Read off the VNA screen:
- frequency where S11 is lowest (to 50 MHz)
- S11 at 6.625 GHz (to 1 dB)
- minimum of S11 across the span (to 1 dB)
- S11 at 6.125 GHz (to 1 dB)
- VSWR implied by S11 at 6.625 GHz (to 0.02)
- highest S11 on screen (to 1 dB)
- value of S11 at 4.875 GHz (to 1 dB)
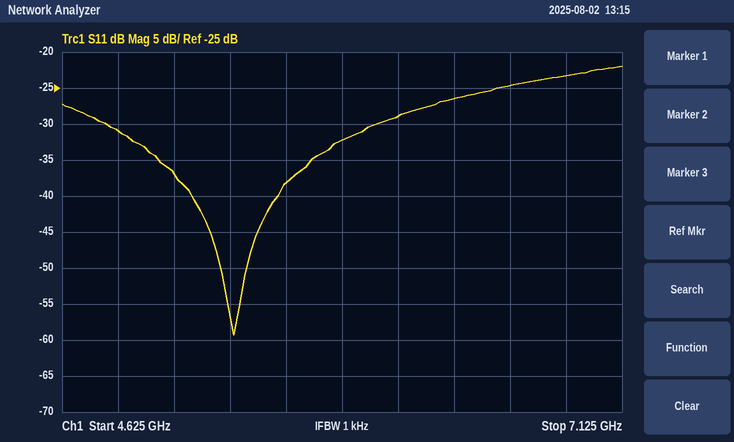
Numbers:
5.40 GHz
-25 dB
-59 dB
-29 dB
1.12
-22 dB
-31 dB
